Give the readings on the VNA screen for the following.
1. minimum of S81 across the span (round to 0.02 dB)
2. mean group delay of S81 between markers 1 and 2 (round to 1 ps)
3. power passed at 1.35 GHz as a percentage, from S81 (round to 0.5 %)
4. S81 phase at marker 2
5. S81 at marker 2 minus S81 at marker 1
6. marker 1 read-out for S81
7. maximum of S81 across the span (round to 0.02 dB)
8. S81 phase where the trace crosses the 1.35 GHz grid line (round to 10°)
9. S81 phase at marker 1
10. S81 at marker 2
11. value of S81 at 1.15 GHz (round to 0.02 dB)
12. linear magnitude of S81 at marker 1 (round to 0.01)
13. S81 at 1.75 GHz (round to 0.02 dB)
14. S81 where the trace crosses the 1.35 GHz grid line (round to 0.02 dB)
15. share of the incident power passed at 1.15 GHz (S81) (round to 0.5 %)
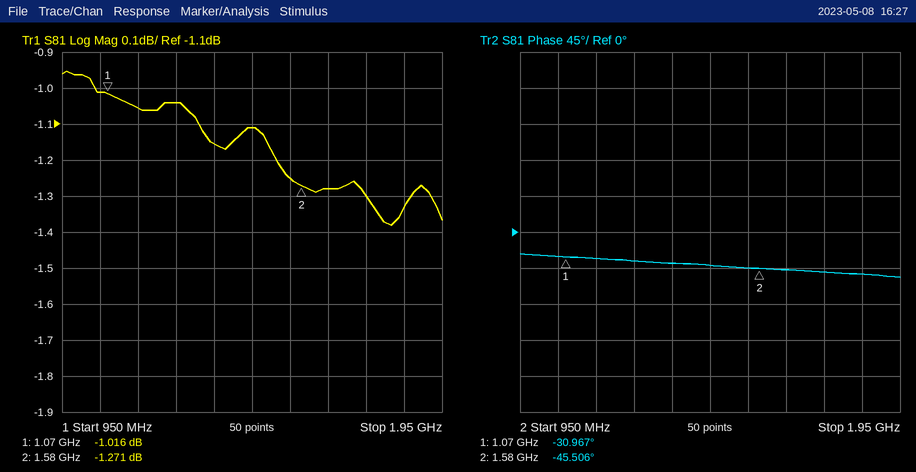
-1.38 dB
79 ps
76.5 %
-45.506°
-0.255 dB
-1.016 dB
-0.96 dB
-40°
-30.967°
-1.271 dB
-1.06 dB
0.89
-1.30 dB
-1.16 dB
78.5 %
